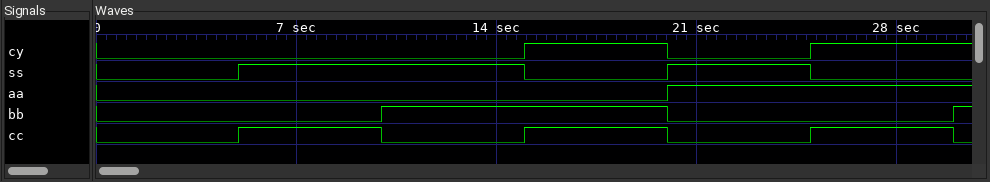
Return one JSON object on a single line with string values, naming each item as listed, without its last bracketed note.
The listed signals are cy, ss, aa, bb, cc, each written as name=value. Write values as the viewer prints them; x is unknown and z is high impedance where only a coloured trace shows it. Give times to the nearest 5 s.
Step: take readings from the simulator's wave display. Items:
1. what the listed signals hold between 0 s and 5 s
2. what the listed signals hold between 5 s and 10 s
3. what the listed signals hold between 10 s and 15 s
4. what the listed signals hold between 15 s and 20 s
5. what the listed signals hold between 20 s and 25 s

{"what the listed signals hold between 0 s and 5 s": "cy=0, ss=0, aa=0, bb=0, cc=0", "what the listed signals hold between 5 s and 10 s": "cy=0, ss=1, aa=0, bb=0, cc=1", "what the listed signals hold between 10 s and 15 s": "cy=0, ss=1, aa=0, bb=1, cc=0", "what the listed signals hold between 15 s and 20 s": "cy=1, ss=0, aa=0, bb=1, cc=1", "what the listed signals hold between 20 s and 25 s": "cy=0, ss=1, aa=1, bb=0, cc=0"}
